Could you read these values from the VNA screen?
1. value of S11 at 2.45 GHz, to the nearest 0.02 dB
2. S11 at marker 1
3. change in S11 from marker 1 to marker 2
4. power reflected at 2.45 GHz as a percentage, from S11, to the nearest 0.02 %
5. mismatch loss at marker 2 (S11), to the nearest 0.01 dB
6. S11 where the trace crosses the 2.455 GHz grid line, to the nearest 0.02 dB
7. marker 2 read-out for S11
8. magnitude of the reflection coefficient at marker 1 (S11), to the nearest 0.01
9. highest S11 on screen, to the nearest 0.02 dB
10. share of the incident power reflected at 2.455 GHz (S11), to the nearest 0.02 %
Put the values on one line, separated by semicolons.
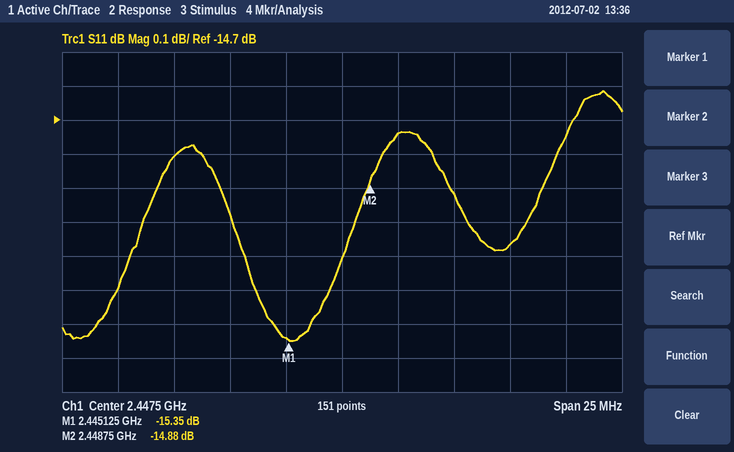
-14.74 dB; -15.35 dB; 0.47 dB; 3.36 %; 0.14 dB; -15.06 dB; -14.88 dB; 0.17; -14.62 dB; 3.12 %
